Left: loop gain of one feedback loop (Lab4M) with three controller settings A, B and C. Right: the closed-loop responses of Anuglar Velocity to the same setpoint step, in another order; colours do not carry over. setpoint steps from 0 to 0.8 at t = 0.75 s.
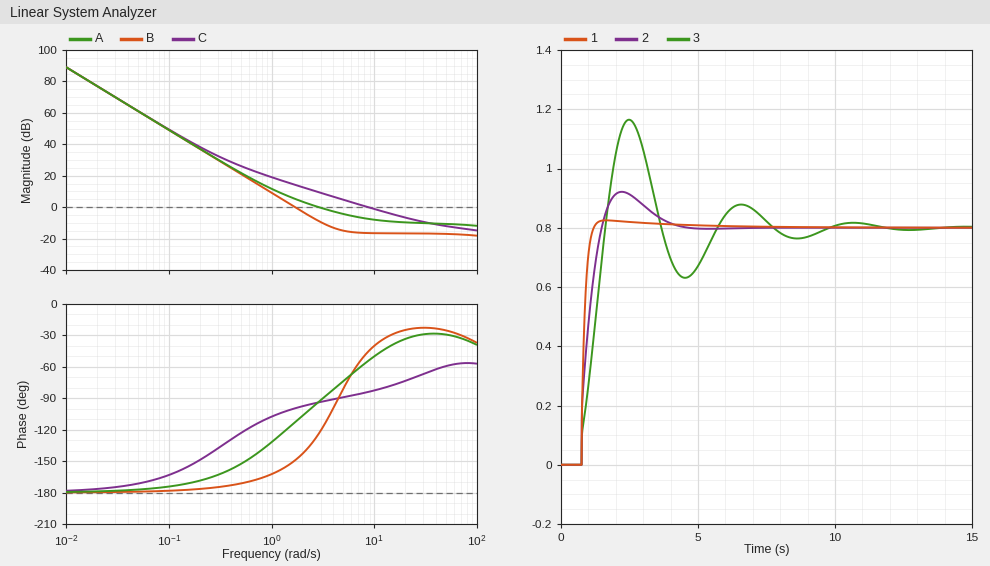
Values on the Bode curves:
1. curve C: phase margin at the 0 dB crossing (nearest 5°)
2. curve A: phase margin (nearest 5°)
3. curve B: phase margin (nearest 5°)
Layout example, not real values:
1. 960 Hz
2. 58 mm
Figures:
1. 95°
2. 85°
3. 30°
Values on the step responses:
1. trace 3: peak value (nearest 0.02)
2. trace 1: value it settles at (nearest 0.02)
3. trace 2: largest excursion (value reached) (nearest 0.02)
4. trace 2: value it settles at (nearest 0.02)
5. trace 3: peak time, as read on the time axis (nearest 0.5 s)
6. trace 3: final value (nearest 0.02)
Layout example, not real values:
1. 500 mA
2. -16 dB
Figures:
1. 1.16
2. 0.80
3. 0.92
4. 0.80
5. 2.5 s
6. 0.80
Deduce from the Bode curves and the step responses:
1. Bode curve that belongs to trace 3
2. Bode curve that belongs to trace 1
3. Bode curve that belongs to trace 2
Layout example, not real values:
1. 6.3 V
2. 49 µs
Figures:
1. B
2. C
3. A
